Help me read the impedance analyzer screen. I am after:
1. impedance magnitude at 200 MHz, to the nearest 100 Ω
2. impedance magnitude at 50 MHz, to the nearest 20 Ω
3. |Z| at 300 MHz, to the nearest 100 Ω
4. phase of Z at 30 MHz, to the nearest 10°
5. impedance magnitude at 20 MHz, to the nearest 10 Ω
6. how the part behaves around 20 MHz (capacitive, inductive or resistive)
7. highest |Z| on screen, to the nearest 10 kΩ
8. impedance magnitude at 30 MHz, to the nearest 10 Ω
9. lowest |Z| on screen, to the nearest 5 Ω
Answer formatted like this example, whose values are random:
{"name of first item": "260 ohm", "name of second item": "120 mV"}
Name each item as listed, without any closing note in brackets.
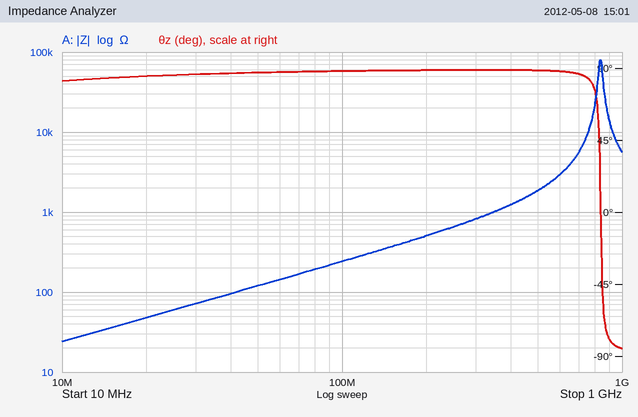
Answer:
{"impedance magnitude at 200 MHz, to the nearest 100 Ω": "500 Ω", "impedance magnitude at 50 MHz, to the nearest 20 Ω": "120 Ω", "|Z| at 300 MHz, to the nearest 100 Ω": "800 Ω", "phase of Z at 30 MHz, to the nearest 10°": "90°", "impedance magnitude at 20 MHz, to the nearest 10 Ω": "50 Ω", "how the part behaves around 20 MHz": "inductive", "highest |Z| on screen, to the nearest 10 kΩ": "80 kΩ", "impedance magnitude at 30 MHz, to the nearest 10 Ω": "70 Ω", "lowest |Z| on screen, to the nearest 5 Ω": "25 Ω"}
